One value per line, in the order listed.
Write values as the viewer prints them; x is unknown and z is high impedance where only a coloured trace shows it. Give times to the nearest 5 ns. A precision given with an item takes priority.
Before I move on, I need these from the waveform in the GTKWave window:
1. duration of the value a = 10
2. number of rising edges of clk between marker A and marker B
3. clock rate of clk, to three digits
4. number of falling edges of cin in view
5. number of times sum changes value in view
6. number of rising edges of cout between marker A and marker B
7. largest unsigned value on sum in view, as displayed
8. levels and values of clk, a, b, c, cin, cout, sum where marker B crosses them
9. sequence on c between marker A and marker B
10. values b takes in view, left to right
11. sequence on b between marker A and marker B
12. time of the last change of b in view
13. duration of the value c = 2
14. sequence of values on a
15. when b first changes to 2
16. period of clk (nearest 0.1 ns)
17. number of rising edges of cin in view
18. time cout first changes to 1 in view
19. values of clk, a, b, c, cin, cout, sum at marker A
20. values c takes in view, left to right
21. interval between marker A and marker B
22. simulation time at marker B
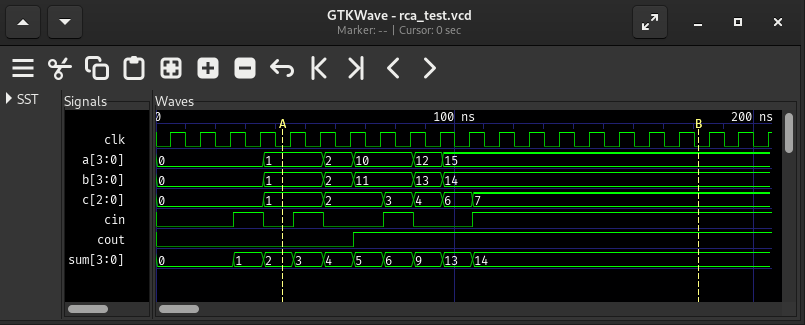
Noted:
20 ns
14
100 MHz
3
9
1
14
clk=0, a=15, b=14, c=7, cin=1, cout=1, sum=14
1, 2, 3, 4, 6, 7
0, 1, 2, 11, 13, 14
1, 2, 11, 13, 14
95 ns
20 ns
0, 1, 2, 10, 12, 15
55 ns
10 ns
4
65 ns
clk=0, a=1, b=1, c=1, cin=0, cout=0, sum=2
0, 1, 2, 3, 4, 6, 7
140 ns
180 ns
